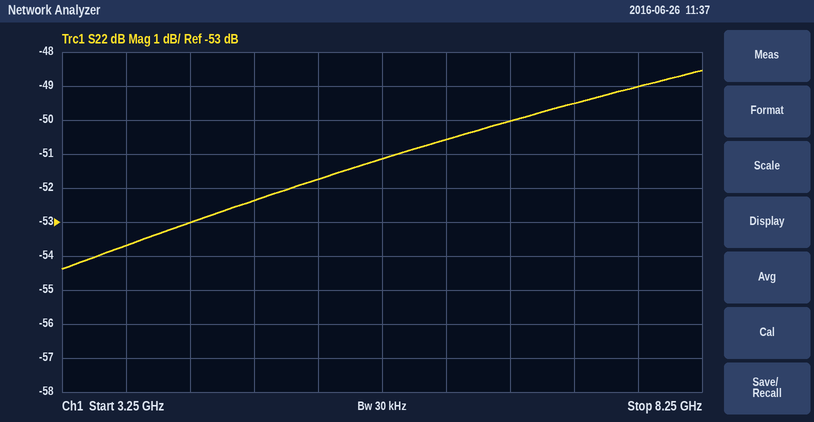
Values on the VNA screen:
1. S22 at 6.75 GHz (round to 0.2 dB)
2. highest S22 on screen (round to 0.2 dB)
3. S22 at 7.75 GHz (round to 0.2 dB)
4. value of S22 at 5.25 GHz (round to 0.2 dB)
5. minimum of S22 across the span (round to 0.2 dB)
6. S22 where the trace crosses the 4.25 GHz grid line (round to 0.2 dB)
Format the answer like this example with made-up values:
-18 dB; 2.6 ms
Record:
-50.0 dB; -48.6 dB; -49.0 dB; -51.8 dB; -54.4 dB; -53.0 dB
